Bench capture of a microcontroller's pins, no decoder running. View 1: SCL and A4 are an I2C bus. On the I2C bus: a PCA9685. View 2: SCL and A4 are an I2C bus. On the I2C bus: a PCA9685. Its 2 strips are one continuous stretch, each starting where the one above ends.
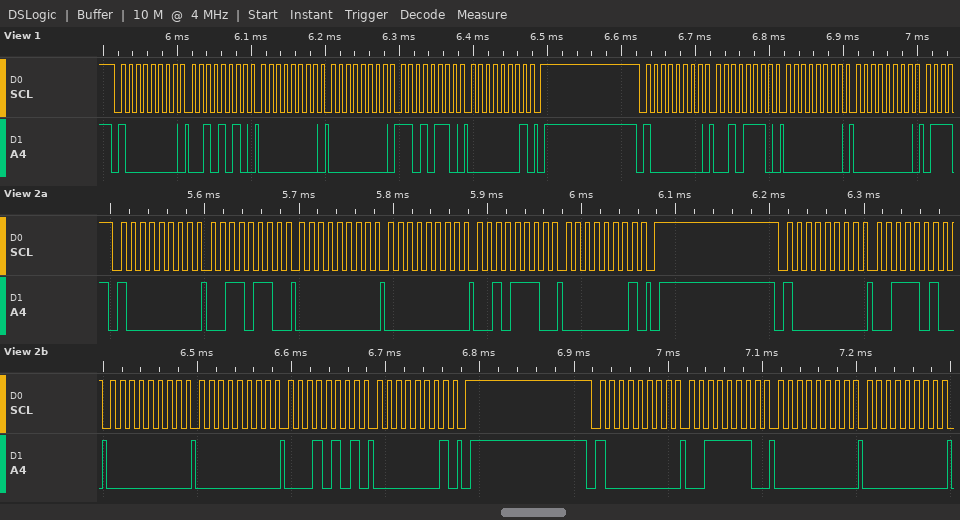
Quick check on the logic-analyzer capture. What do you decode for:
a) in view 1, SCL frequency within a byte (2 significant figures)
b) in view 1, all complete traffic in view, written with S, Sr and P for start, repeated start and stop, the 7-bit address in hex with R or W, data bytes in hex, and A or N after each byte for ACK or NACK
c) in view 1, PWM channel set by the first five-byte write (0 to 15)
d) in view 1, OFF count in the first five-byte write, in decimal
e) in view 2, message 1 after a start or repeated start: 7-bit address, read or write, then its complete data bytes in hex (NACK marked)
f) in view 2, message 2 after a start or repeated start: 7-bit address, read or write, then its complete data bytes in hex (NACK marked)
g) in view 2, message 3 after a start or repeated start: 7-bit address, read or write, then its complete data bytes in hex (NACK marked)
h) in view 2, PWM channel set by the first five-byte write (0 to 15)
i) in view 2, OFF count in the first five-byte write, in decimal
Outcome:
100 kHz
S 40W A 2A A 00 A 00 A D6 A 01 A P S 40W A 2E A 00 A 00 A
9
470
0x40 write: 36 00 00 2E 01
0x40 write: 3A 00 00 15 01
0x40 write: 3E 00 00
12
302
